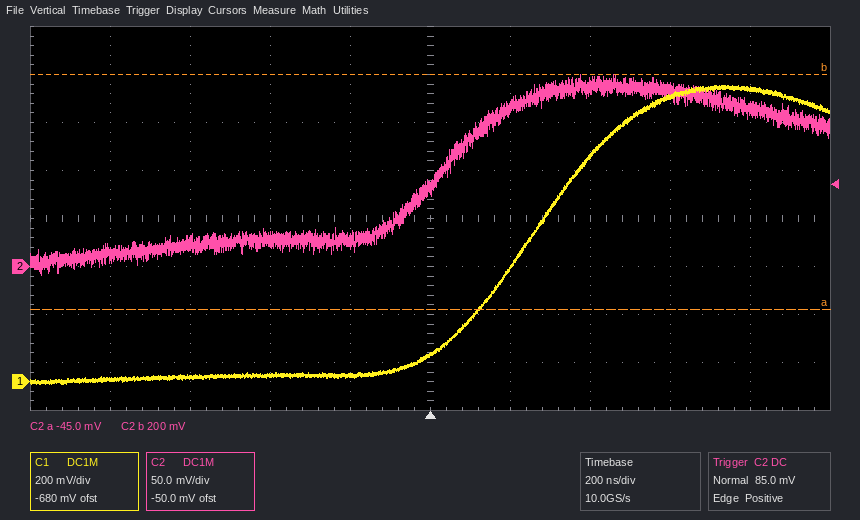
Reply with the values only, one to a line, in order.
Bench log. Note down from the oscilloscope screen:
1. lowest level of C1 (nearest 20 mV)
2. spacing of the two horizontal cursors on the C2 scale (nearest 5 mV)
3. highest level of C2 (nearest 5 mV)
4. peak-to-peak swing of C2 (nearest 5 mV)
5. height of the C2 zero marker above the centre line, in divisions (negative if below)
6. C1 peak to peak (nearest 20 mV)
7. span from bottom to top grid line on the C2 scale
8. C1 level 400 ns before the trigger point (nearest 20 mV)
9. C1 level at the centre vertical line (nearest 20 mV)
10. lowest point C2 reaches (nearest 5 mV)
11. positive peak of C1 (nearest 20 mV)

0 mV
245 mV
200 mV
210 mV
-1.0 div
1.24 V
400 mV
20 mV
120 mV
-10 mV
1.24 V
